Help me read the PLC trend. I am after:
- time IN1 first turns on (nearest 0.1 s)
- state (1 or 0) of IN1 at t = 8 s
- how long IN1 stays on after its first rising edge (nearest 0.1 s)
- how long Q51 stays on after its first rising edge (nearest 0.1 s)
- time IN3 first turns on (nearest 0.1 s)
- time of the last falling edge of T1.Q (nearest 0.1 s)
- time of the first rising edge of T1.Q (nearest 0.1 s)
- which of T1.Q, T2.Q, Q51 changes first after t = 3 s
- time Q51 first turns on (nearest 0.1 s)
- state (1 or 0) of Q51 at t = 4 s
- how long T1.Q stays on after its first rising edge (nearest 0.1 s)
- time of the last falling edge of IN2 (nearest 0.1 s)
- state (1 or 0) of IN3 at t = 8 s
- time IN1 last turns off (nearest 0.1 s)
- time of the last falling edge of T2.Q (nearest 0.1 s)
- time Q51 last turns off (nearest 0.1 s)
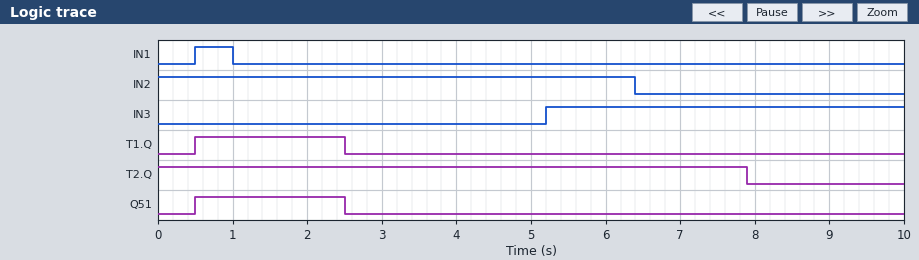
0.5 s
0
0.5 s
2.0 s
5.2 s
2.5 s
0.5 s
T2.Q
0.5 s
0
2.0 s
6.4 s
1
1.0 s
7.9 s
2.5 s
